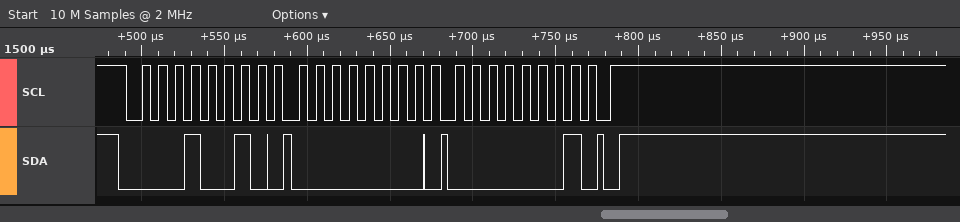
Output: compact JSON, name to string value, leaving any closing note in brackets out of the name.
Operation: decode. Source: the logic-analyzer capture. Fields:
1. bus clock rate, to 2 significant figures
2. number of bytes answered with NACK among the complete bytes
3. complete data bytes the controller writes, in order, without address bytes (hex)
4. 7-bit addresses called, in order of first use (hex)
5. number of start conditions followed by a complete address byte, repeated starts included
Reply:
{"bus clock rate, to 2 significant figures": "100 kHz", "number of bytes answered with NACK among the complete bytes": "0", "complete data bytes the controller writes, in order, without address bytes": "00 01", "7-bit addresses called, in order of first use": "0x09", "number of start conditions followed by a complete address byte, repeated starts included": "1"}
